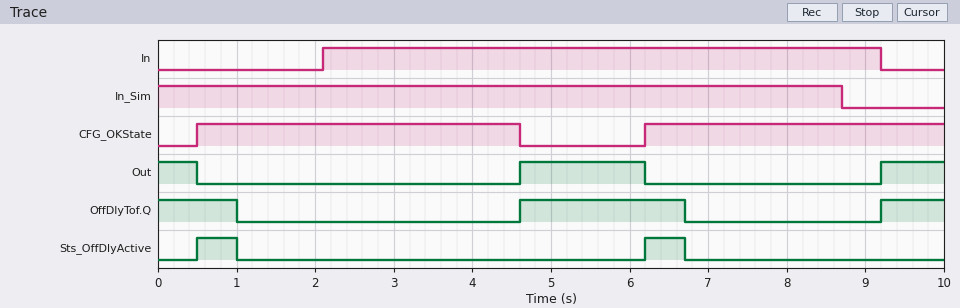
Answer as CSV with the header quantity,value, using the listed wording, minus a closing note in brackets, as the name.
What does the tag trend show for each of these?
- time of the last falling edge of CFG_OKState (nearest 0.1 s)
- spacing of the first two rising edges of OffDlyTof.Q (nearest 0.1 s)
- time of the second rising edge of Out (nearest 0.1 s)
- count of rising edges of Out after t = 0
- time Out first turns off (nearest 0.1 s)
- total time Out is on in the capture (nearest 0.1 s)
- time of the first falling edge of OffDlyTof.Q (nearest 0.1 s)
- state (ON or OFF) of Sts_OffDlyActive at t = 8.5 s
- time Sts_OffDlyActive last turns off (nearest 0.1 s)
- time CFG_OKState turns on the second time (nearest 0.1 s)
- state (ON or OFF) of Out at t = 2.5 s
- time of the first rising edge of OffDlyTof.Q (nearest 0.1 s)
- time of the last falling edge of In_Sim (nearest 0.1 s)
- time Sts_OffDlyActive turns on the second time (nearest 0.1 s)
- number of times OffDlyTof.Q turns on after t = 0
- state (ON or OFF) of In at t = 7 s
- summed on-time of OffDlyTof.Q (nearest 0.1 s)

quantity,value
time of the last falling edge of CFG_OKState,4.6 s
spacing of the first two rising edges of OffDlyTof.Q,4.6 s
time of the second rising edge of Out,9.2 s
count of rising edges of Out after t = 0,2
time Out first turns off,0.5 s
total time Out is on in the capture,2.9 s
time of the first falling edge of OffDlyTof.Q,1.0 s
state (ON or OFF) of Sts_OffDlyActive at t = 8.5 s,OFF
time Sts_OffDlyActive last turns off,6.7 s
time CFG_OKState turns on the second time,6.2 s
state (ON or OFF) of Out at t = 2.5 s,OFF
time of the first rising edge of OffDlyTof.Q,4.6 s
time of the last falling edge of In_Sim,8.7 s
time Sts_OffDlyActive turns on the second time,6.2 s
number of times OffDlyTof.Q turns on after t = 0,2
state (ON or OFF) of In at t = 7 s,ON
summed on-time of OffDlyTof.Q,3.9 s
